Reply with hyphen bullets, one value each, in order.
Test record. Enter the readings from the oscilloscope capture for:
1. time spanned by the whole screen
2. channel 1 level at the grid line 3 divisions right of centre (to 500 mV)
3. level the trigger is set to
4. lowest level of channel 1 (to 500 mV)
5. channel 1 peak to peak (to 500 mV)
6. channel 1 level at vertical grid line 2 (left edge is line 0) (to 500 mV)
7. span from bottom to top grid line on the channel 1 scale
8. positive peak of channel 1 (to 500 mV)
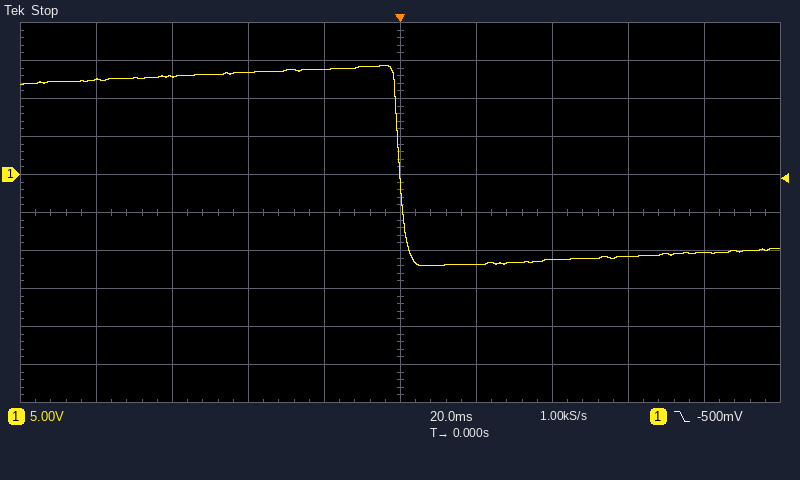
- 200 ms
- -11.0 V
- -500 mV
- -12.0 V
- 26.5 V
- 13.0 V
- 50 V
- 14.5 V
